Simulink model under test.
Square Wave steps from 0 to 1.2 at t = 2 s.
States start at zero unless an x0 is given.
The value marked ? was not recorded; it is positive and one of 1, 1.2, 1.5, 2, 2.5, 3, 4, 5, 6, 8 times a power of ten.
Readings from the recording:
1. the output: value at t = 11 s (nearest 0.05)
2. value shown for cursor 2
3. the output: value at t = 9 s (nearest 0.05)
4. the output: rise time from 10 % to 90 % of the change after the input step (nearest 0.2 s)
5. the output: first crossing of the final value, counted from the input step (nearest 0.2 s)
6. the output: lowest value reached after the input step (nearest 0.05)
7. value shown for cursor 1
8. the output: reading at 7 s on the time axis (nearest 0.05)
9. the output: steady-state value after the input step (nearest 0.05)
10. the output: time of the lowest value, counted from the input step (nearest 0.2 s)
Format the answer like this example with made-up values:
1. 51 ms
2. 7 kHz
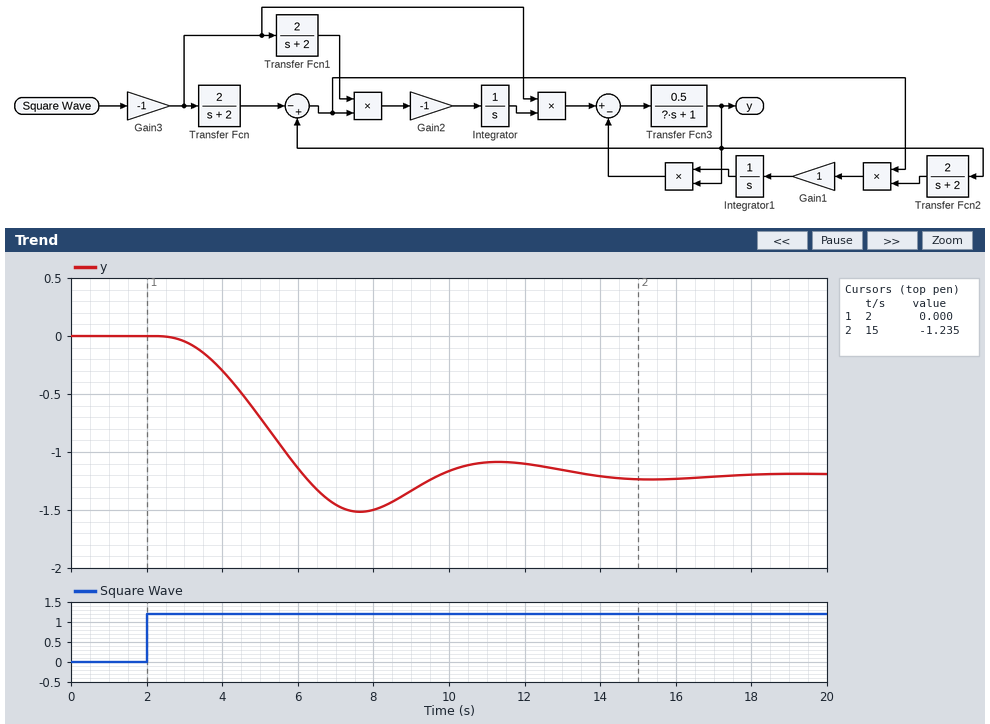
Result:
1. -1.10
2. -1.235
3. -1.35
4. 2.4 s
5. 4.2 s
6. -1.50
7. 0.000
8. -1.45
9. -1.20
10. 5.6 s
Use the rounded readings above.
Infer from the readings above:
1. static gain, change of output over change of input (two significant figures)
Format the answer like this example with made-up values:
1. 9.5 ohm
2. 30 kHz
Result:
1. -1.0
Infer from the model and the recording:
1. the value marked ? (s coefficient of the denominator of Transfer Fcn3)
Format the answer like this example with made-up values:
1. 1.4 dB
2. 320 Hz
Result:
1. 2
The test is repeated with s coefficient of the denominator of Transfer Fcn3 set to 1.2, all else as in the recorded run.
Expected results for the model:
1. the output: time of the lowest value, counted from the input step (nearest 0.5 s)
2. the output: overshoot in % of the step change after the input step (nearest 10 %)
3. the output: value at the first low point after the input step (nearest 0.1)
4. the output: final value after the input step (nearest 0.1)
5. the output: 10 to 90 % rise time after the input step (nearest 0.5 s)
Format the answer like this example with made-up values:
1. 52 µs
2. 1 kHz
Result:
1. 5.0 s
2. 20 %
3. -1.4
4. -1.2
5. 2.0 s
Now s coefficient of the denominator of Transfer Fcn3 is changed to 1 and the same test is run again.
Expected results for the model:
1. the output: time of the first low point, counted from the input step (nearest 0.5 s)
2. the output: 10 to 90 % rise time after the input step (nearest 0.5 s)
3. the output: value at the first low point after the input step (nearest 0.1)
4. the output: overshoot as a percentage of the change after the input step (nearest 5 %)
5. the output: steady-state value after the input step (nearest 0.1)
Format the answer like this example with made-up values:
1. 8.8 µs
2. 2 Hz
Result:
1. 4.5 s
2. 2.0 s
3. -1.4
4. 15 %
5. -1.2
